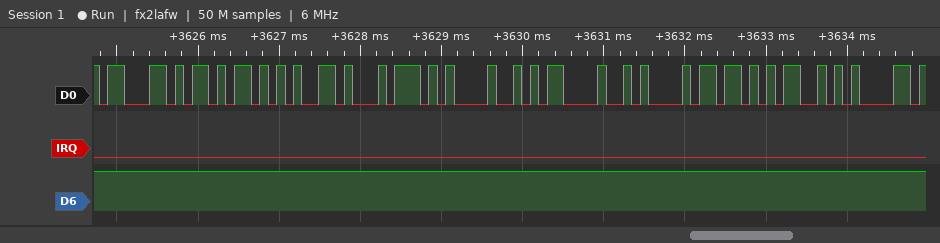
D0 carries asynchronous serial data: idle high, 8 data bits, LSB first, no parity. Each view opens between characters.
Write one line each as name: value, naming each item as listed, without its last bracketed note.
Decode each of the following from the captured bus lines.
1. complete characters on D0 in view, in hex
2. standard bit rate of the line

complete characters on D0 in view, in hex: 63, 6B, 65, 74, 21, 0D, 0A, 5B, 53
standard bit rate of the line: 9600 baud
